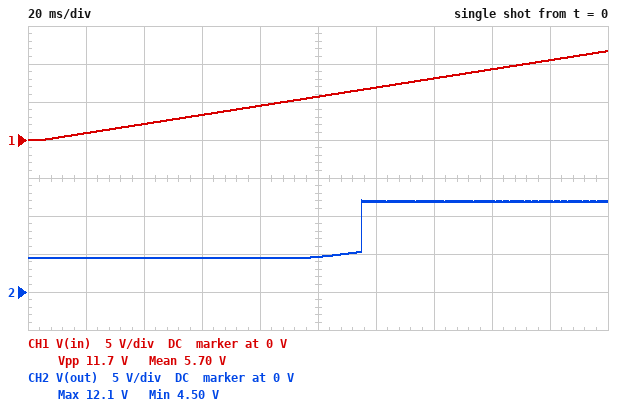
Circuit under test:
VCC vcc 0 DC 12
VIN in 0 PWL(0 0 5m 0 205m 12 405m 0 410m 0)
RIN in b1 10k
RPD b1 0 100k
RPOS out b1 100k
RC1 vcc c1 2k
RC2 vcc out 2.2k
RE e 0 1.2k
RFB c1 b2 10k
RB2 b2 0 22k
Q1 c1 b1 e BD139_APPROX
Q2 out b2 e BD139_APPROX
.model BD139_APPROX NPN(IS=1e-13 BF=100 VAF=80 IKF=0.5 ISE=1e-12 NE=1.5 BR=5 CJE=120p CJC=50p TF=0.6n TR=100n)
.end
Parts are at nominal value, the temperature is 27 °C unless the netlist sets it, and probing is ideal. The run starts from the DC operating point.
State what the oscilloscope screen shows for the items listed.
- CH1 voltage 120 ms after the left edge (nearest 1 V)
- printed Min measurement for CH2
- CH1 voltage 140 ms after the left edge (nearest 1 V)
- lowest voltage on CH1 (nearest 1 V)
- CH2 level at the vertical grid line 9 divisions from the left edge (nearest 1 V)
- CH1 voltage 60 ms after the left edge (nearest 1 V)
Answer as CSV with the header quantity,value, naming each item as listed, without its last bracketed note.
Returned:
quantity,value
CH1 voltage 120 ms after the left edge,7 V
printed Min measurement for CH2,4.50 V
CH1 voltage 140 ms after the left edge,8 V
lowest voltage on CH1,0 V
CH2 level at the vertical grid line 9 divisions from the left edge,12 V
CH1 voltage 60 ms after the left edge,3 V
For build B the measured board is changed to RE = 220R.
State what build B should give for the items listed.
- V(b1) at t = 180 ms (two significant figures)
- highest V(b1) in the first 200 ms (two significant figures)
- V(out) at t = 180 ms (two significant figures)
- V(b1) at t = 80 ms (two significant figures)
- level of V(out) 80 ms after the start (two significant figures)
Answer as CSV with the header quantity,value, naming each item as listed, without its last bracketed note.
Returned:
quantity,value
V(b1) at t = 180 ms,2.0 V
highest V(b1) in the first 200 ms,2.5 V
V(out) at t = 180 ms,12 V
V(b1) at t = 80 ms,1.9 V
level of V(out) 80 ms after the start,12 V
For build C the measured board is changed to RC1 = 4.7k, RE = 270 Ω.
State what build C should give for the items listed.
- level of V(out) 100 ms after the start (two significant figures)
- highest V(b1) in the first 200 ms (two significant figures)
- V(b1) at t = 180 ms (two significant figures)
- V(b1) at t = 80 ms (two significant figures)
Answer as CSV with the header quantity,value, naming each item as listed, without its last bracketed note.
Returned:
quantity,value
level of V(out) 100 ms after the start,12 V
highest V(b1) in the first 200 ms,2.3 V
V(b1) at t = 180 ms,1.5 V
V(b1) at t = 80 ms,1.4 V
